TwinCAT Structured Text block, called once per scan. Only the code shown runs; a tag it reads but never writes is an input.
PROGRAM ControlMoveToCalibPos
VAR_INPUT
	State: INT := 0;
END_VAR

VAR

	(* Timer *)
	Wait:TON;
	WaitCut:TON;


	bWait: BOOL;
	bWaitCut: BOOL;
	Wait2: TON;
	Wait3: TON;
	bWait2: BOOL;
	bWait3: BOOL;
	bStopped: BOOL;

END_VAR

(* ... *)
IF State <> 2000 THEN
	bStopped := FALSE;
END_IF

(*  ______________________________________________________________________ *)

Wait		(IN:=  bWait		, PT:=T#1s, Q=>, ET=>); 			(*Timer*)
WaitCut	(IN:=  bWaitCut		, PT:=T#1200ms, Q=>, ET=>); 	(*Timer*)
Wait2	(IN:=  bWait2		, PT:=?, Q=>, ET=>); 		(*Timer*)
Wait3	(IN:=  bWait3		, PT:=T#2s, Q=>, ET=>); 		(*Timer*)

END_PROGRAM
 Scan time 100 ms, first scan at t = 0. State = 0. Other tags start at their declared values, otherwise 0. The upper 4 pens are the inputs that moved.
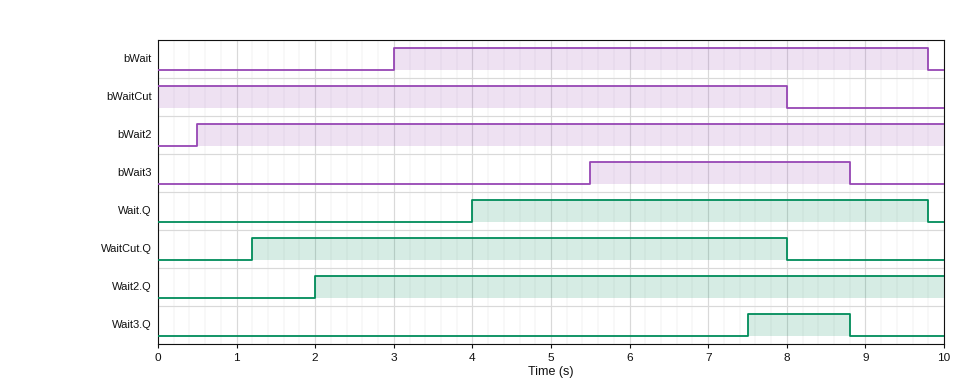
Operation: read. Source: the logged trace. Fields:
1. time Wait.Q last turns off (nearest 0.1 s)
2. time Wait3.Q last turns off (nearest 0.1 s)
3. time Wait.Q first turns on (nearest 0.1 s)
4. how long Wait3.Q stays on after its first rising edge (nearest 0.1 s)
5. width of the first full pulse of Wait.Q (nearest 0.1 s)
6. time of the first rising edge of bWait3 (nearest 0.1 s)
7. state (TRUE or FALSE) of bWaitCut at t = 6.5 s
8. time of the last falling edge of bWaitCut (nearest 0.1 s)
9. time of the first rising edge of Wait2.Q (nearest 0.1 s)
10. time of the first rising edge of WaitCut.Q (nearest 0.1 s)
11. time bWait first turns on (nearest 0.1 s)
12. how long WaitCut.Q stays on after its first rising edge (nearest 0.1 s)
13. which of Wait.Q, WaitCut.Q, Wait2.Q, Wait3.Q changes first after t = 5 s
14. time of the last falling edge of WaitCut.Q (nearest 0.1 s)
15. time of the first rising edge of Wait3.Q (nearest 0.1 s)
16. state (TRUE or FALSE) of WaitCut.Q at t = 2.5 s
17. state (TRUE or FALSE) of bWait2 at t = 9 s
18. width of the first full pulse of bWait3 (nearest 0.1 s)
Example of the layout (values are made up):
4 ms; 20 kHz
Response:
9.8 s; 8.8 s; 4.0 s; 1.3 s; 5.8 s; 5.5 s; TRUE; 8.0 s; 2.0 s; 1.2 s; 3.0 s; 6.8 s; Wait3.Q; 8.0 s; 7.5 s; TRUE; TRUE; 3.3 s
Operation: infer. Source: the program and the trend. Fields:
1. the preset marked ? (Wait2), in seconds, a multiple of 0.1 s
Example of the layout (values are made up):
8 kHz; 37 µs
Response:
1.5 s
